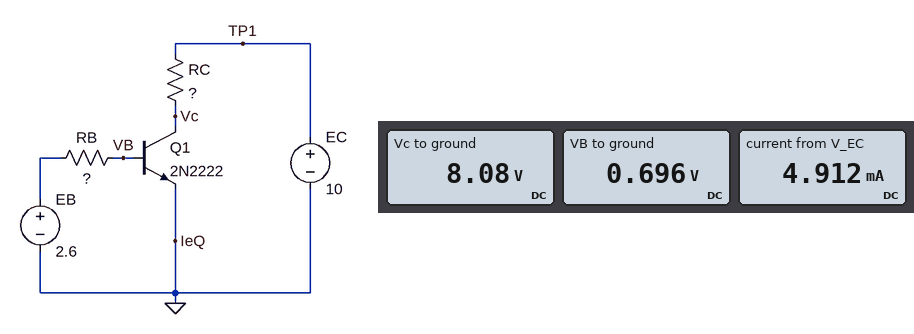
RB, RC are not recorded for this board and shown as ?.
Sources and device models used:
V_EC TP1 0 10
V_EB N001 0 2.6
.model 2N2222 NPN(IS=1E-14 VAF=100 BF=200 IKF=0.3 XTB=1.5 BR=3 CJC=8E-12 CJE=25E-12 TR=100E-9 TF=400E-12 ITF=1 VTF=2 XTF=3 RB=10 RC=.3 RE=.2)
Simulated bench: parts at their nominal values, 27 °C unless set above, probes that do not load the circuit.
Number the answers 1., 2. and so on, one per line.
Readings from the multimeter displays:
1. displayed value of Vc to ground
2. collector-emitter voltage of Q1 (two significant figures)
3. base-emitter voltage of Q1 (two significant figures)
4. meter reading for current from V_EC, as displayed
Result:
1. 8.08 V
2. 8.1 V
3. 700 mV
4. 4.912 mA
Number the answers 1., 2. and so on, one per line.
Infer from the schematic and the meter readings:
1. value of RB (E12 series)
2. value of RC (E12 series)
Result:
1. 82 kΩ
2. 390 Ω
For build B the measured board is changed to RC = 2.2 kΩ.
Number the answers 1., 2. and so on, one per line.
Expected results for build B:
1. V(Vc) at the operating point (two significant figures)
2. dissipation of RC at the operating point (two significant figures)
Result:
1. 210 mV
2. 44 mW
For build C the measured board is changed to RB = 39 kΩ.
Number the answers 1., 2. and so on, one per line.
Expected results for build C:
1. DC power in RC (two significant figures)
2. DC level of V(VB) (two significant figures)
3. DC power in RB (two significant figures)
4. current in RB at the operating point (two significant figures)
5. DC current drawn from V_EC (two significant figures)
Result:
1. 38 mW
2. 720 mV
3. 91 µW
4. 48 µA
5. 9.9 mA
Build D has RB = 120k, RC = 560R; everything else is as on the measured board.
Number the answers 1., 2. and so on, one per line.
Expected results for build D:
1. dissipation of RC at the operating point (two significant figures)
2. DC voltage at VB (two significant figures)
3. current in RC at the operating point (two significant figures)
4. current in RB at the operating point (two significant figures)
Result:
1. 6.4 mW
2. 690 mV
3. 3.4 mA
4. 16 µA
